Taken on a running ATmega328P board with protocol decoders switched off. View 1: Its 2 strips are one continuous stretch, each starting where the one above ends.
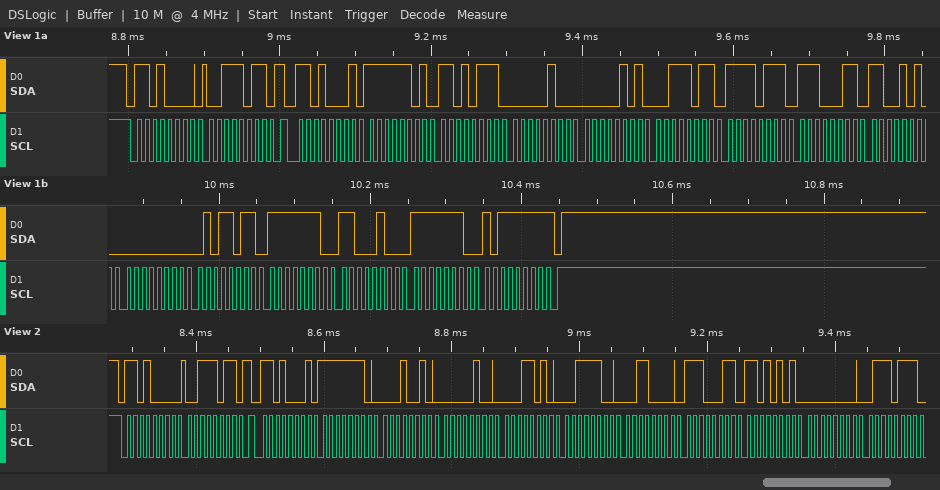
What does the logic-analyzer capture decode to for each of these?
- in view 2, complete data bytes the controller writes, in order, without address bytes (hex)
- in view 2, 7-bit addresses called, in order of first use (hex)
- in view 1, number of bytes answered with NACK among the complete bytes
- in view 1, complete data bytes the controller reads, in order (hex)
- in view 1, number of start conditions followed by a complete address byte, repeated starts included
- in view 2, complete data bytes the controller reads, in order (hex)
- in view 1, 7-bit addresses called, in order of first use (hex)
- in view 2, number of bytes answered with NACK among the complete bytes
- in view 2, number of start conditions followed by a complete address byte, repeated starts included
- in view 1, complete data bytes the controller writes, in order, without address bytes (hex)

3B
0x68
1
FD D7 04 05 3B F7 E3 CA 00 5B FE C4 FE BF
2
FE 12 04 1A 3C 30 E3 D5 00 77
0x68
0
2
3B
